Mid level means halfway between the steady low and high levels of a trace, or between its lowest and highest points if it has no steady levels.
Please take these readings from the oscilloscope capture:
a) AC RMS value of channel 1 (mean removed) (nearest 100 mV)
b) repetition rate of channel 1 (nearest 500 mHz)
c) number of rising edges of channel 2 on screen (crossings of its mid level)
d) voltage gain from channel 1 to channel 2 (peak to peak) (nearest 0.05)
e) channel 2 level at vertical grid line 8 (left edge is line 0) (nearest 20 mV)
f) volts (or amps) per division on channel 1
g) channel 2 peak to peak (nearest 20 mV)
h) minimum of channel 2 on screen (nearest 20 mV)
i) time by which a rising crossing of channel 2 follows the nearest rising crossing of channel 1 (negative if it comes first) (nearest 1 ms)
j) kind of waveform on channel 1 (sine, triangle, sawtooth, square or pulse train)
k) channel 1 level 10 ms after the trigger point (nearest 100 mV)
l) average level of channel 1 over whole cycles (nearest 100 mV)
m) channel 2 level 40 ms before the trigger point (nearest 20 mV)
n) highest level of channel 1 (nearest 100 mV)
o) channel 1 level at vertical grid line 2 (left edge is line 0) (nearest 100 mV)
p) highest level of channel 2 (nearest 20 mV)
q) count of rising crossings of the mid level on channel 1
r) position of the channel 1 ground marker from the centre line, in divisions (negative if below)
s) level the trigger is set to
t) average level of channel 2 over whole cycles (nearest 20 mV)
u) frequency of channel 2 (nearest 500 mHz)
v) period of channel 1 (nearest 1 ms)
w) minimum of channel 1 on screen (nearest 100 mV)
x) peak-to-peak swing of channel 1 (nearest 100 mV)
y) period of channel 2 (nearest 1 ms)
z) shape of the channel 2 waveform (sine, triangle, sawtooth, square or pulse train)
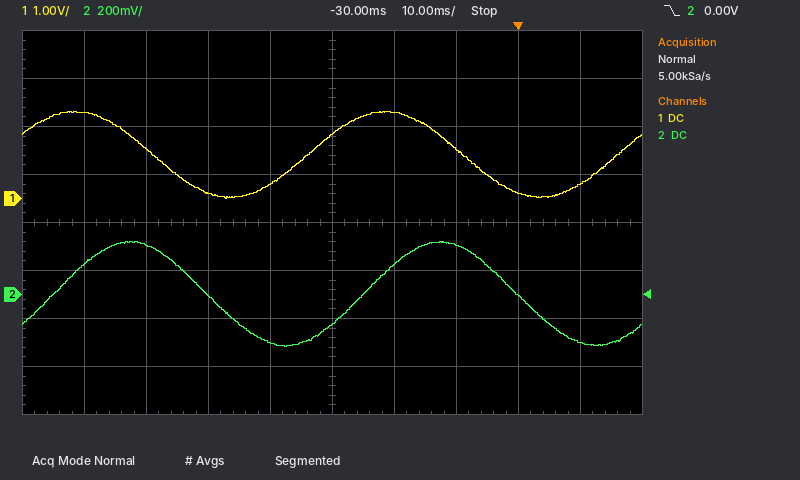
600 mV
20.0 Hz
2
0.25
0 mV
1 V
440 mV
-220 mV
+9 ms
sine
300 mV
900 mV
-200 mV
1.8 V
1.0 V
220 mV
2
+0.5 div
0.00 V
0 mV
20.0 Hz
50 ms
0.0 V
1.8 V
50 ms
sine
